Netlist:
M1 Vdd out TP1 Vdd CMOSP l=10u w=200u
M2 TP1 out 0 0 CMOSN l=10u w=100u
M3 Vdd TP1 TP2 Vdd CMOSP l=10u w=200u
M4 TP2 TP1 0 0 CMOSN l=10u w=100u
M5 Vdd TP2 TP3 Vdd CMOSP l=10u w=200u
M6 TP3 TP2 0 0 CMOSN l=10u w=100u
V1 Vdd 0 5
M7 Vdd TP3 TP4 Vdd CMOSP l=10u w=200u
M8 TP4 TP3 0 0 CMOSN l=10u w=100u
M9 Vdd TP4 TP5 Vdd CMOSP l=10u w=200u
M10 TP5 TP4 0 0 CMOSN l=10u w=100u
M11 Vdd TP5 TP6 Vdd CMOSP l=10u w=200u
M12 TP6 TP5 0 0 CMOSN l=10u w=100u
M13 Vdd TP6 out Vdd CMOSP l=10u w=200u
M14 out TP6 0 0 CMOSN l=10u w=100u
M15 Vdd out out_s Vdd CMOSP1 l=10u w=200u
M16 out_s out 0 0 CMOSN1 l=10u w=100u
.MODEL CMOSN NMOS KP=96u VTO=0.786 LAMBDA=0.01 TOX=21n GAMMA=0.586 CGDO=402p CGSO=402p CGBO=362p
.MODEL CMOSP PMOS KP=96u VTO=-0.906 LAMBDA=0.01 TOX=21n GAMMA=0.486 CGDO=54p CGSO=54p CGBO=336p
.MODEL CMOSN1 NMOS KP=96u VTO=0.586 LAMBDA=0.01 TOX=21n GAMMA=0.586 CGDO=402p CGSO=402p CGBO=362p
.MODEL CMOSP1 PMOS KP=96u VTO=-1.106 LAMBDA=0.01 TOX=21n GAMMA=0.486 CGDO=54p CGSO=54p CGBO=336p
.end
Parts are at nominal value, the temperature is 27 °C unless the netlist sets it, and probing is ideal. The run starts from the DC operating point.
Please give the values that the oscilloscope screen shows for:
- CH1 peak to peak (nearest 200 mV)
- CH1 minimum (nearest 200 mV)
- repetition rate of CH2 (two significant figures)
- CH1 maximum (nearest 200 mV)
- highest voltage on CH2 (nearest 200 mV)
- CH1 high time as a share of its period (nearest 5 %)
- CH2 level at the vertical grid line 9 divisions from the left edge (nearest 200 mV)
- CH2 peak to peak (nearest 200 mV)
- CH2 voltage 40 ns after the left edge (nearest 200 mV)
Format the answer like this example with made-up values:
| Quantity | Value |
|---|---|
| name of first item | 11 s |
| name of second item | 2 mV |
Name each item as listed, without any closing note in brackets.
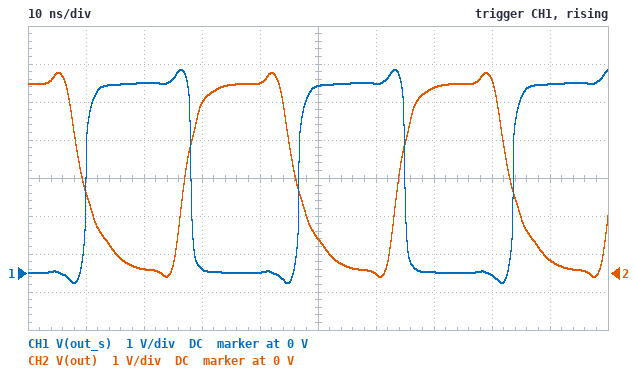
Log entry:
| Quantity | Value |
|---|---|
| CH1 peak to peak | 5.6 V |
| CH1 minimum | -200 mV |
| repetition rate of CH2 | 27 MHz |
| CH1 maximum | 5.4 V |
| highest voltage on CH2 | 5.2 V |
| CH1 high time as a share of its period | 50 % |
| CH2 level at the vertical grid line 9 divisions from the left edge | 400 mV |
| CH2 peak to peak | 5.4 V |
| CH2 voltage 40 ns after the left edge | 5.0 V |
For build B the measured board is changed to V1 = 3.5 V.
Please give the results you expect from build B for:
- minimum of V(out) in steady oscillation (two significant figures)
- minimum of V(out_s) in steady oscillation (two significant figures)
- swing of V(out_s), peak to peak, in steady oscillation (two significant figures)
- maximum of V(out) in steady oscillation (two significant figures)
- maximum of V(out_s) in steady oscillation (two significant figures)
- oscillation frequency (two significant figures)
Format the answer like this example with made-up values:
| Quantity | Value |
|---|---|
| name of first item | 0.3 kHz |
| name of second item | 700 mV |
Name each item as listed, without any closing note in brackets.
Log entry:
| Quantity | Value |
|---|---|
| minimum of V(out) in steady oscillation | -96 mV |
| minimum of V(out_s) in steady oscillation | -200 mV |
| swing of V(out_s), peak to peak, in steady oscillation | 4.0 V |
| maximum of V(out) in steady oscillation | 3.7 V |
| maximum of V(out_s) in steady oscillation | 3.8 V |
| oscillation frequency | 16 MHz |
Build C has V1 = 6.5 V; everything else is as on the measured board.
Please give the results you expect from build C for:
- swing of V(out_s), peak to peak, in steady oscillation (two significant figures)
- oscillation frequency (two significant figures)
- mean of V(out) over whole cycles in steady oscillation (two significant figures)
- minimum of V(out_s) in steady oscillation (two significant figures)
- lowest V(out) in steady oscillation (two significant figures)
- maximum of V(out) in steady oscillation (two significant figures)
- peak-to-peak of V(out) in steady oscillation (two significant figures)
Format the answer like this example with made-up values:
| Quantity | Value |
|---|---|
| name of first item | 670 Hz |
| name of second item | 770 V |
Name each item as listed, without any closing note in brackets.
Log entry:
| Quantity | Value |
|---|---|
| swing of V(out_s), peak to peak, in steady oscillation | 7.3 V |
| oscillation frequency | 39 MHz |
| mean of V(out) over whole cycles in steady oscillation | 3.5 V |
| minimum of V(out_s) in steady oscillation | -330 mV |
| lowest V(out) in steady oscillation | -110 mV |
| maximum of V(out) in steady oscillation | 6.8 V |
| peak-to-peak of V(out) in steady oscillation | 6.9 V |
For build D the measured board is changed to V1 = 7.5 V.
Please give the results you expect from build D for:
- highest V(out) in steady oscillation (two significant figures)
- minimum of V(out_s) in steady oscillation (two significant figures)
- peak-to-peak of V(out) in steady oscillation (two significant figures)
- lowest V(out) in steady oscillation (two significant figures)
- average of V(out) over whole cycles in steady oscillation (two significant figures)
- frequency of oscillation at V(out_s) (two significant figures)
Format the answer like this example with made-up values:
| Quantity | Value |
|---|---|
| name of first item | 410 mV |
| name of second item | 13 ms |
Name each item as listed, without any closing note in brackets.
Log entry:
| Quantity | Value |
|---|---|
| highest V(out) in steady oscillation | 7.9 V |
| minimum of V(out_s) in steady oscillation | -370 mV |
| peak-to-peak of V(out) in steady oscillation | 8.0 V |
| lowest V(out) in steady oscillation | -110 mV |
| average of V(out) over whole cycles in steady oscillation | 4.0 V |
| frequency of oscillation at V(out_s) | 47 MHz |
